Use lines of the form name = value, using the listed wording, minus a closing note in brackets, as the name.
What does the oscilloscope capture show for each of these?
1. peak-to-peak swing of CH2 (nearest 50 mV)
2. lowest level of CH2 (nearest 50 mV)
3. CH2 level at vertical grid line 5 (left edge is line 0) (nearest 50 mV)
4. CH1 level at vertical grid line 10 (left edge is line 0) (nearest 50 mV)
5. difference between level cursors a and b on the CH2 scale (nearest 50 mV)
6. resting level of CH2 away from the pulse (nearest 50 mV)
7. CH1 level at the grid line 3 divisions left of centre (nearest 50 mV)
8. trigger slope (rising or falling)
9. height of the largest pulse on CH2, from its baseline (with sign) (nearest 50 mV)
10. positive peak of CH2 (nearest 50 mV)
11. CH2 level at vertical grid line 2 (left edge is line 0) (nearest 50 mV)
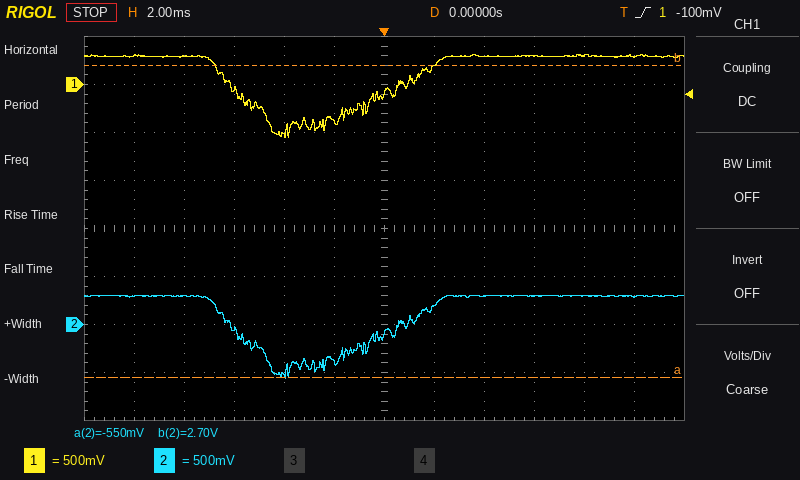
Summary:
peak-to-peak swing of CH2 = 850 mV
lowest level of CH2 = -550 mV
CH2 level at vertical grid line 5 (left edge is line 0) = -400 mV
CH1 level at vertical grid line 10 (left edge is line 0) = 300 mV
difference between level cursors a and b on the CH2 scale = 3.25 V
resting level of CH2 away from the pulse = 300 mV
CH1 level at the grid line 3 divisions left of centre = -50 mV
trigger slope = rising
height of the largest pulse on CH2, from its baseline (with sign) = -850 mV
positive peak of CH2 = 300 mV
CH2 level at vertical grid line 2 (left edge is line 0) = 300 mV
